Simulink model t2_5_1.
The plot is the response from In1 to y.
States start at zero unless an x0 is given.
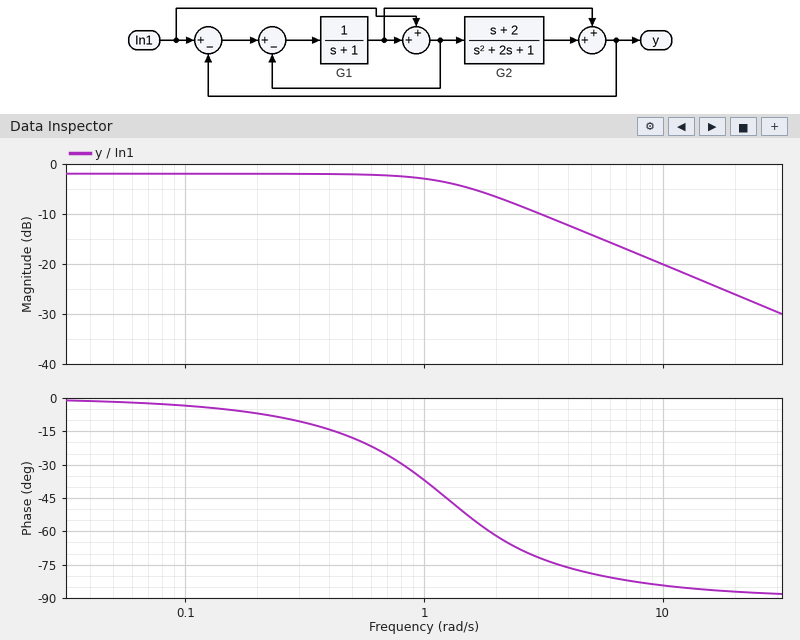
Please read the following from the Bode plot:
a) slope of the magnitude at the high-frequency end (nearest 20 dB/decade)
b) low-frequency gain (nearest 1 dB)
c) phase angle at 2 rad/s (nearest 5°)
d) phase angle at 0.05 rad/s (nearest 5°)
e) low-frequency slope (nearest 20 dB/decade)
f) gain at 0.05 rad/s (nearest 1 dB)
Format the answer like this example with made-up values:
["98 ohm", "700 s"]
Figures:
["-20 dB/decade", "-2 dB", "-60°", "0°", "0 dB/decade", "-2 dB"]
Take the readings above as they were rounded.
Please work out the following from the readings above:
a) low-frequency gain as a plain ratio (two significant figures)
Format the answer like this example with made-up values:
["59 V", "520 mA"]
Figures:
["0.79"]
